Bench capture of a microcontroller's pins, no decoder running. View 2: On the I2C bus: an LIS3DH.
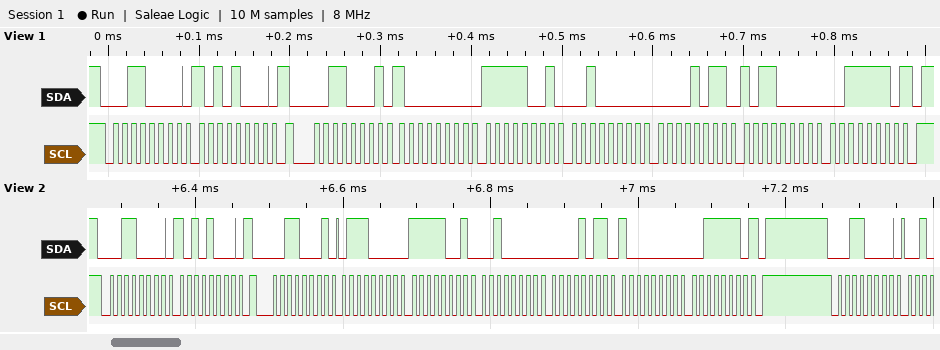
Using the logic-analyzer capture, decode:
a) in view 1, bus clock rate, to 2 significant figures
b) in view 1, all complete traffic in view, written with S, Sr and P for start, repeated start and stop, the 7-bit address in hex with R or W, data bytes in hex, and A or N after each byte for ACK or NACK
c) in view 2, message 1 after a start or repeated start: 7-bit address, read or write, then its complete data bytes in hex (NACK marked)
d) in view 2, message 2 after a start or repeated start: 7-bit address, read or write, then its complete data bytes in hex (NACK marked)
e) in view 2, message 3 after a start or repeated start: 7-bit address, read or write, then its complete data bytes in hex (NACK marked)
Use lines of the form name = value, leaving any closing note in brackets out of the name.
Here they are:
in view 1, bus clock rate, to 2 significant figures = 100 kHz
in view 1, all complete traffic in view, written with S, Sr and P for start, repeated start and stop, the 7-bit address in hex with R or W, data bytes in hex, and A or N after each byte for ACK or NACK = S 18W A A8 A Sr 18R A 80 A F9 A 20 A 0B A B0 A 3E N P
in view 2, message 1 after a start or repeated start: 7-bit address, read or write, then its complete data bytes in hex = 0x18 write: A8
in view 2, message 2 after a start or repeated start: 7-bit address, read or write, then its complete data bytes in hex = 0x18 read: 70 F9 20 0B 80 3E NACK
in view 2, message 3 after a start or repeated start: 7-bit address, read or write, then its complete data bytes in hex = 0x18 write
